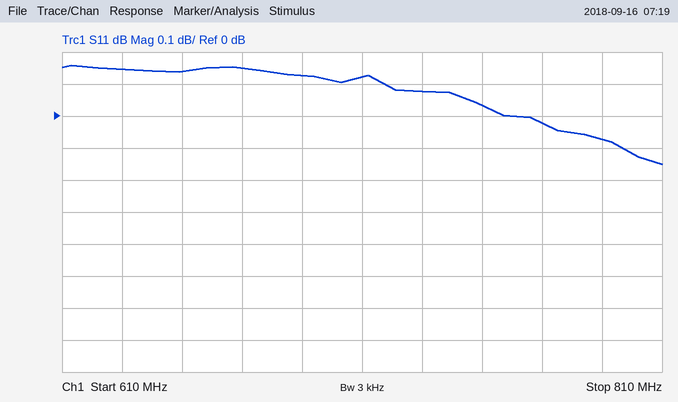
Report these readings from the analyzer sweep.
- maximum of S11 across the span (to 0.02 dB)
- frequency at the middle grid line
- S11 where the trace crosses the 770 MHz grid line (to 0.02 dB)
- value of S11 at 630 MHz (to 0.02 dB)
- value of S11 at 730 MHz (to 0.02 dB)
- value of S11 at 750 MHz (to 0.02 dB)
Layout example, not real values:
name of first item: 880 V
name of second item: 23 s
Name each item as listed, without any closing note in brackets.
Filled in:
maximum of S11 across the span: 0.16 dB
frequency at the middle grid line: 710 MHz
S11 where the trace crosses the 770 MHz grid line: -0.02 dB
value of S11 at 630 MHz: 0.14 dB
value of S11 at 730 MHz: 0.08 dB
value of S11 at 750 MHz: 0.04 dB
